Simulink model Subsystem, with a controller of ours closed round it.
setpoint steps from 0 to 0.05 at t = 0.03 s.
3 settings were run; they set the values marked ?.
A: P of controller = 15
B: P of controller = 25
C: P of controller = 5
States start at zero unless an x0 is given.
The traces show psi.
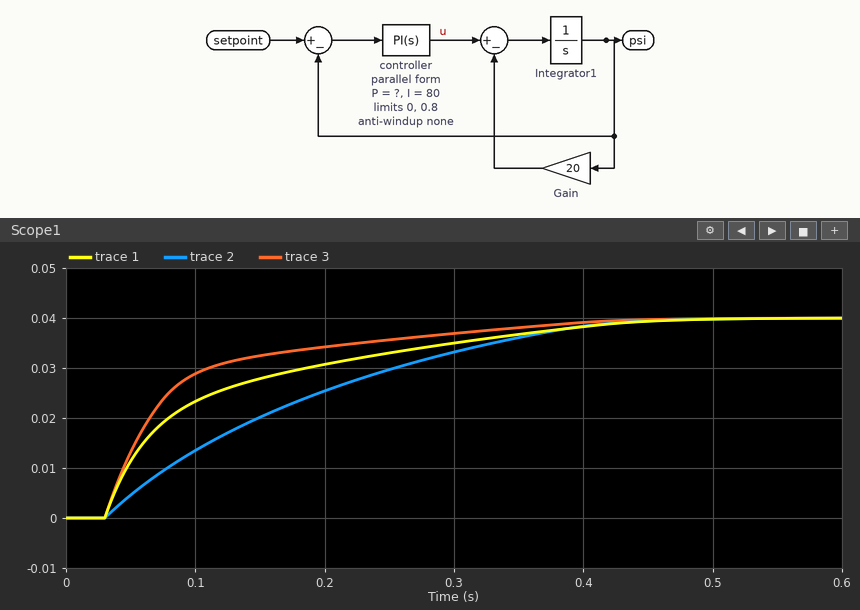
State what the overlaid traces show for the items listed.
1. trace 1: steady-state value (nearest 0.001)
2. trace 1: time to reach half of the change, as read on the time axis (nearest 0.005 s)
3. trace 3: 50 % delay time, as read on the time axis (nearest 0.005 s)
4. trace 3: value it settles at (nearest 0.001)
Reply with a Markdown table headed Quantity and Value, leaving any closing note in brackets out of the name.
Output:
| Quantity | Value |
|---|---|
| trace 1: steady-state value | 0.040 |
| trace 1: time to reach half of the change, as read on the time axis | 0.080 s |
| trace 3: 50 % delay time, as read on the time axis | 0.065 s |
| trace 3: value it settles at | 0.040 |
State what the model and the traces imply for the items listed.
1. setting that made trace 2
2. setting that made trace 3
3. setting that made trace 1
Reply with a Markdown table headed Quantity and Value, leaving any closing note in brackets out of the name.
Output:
| Quantity | Value |
|---|---|
| setting that made trace 2 | C |
| setting that made trace 3 | B |
| setting that made trace 1 | A |
